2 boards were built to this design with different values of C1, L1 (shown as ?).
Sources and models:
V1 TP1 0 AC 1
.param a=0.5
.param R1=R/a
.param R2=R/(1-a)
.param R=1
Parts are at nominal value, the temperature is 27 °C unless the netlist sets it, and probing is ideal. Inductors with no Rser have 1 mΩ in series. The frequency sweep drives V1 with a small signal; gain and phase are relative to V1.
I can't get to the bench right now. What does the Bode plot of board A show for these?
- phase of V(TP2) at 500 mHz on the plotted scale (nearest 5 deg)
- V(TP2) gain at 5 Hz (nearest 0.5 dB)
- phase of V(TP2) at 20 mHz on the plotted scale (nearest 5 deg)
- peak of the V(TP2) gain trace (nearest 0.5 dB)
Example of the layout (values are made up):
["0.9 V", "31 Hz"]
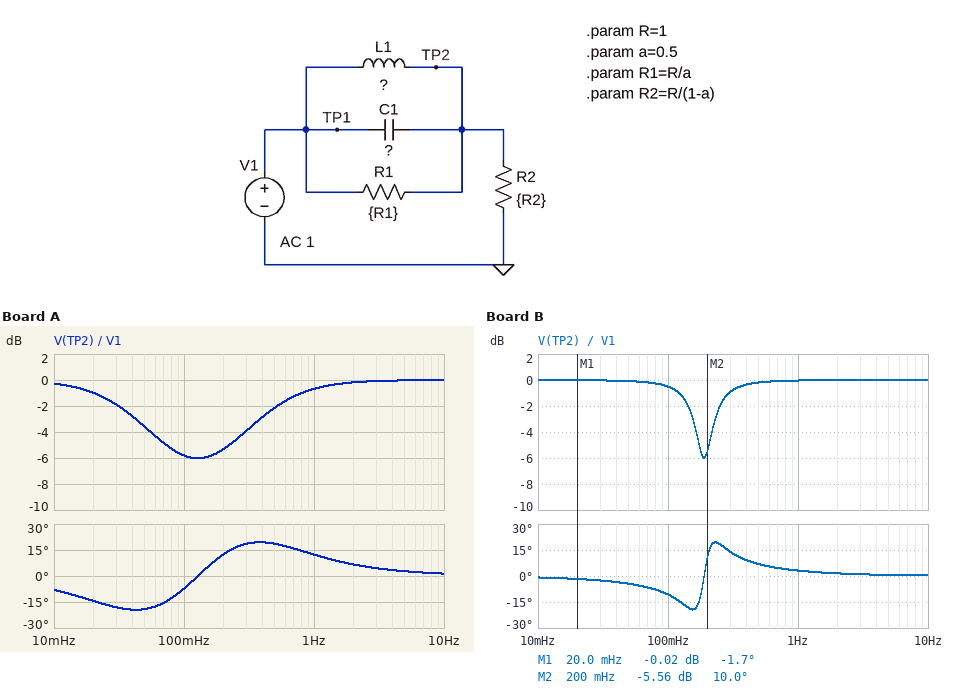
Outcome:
["20 deg", "0 dB", "-15 deg", "0 dB"]
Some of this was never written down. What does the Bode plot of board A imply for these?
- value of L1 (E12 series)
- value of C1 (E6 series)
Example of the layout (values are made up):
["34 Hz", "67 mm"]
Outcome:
["4.7 H", "330 mF"]
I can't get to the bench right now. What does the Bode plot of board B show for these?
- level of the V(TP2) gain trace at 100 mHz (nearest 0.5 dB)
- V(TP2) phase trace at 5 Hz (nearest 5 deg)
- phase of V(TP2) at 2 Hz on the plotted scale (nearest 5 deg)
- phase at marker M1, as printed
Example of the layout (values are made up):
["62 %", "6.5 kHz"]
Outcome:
["-0.5 dB", "0 deg", "0 deg", "-1.7 deg"]
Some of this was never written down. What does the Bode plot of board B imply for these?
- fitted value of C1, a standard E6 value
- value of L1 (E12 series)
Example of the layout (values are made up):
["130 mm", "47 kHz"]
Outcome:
["1.5 F", "470 mH"]
